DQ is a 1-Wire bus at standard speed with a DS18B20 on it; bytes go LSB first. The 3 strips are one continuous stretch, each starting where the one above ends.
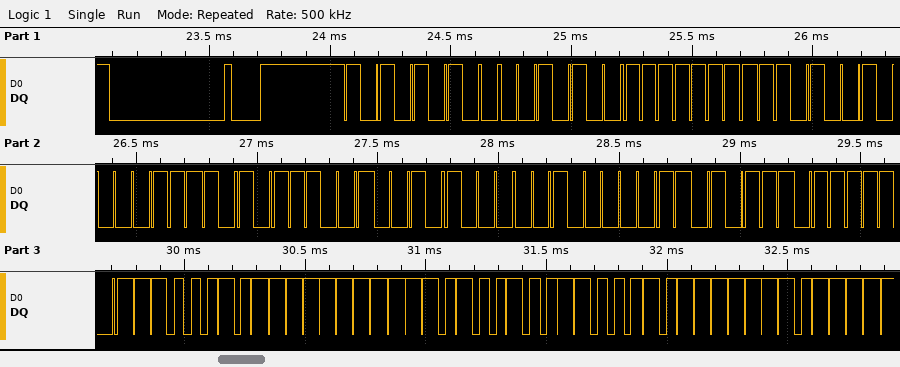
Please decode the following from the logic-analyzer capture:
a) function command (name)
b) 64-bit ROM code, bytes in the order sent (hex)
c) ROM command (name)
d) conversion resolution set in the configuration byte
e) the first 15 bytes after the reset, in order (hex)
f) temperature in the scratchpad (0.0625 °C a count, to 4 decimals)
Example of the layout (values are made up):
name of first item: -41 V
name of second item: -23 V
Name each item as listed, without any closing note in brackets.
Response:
function command: Read Scratchpad
64-bit ROM code, bytes in the order sent: 28 FF 4B 78 9D 14 04 EB
ROM command: Match ROM
conversion resolution set in the configuration byte: 12 bits
the first 15 bytes after the reset, in order: 55 28 FF 4B 78 9D 14 04 EB BE A3 FF 4B 46 7F
temperature in the scratchpad: -5.8125 °C
